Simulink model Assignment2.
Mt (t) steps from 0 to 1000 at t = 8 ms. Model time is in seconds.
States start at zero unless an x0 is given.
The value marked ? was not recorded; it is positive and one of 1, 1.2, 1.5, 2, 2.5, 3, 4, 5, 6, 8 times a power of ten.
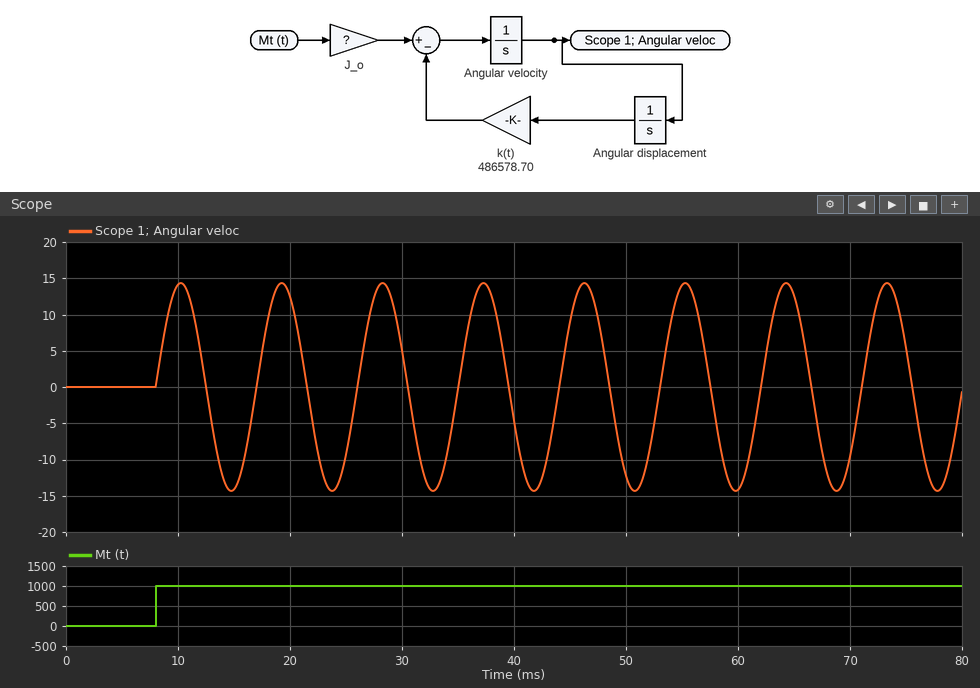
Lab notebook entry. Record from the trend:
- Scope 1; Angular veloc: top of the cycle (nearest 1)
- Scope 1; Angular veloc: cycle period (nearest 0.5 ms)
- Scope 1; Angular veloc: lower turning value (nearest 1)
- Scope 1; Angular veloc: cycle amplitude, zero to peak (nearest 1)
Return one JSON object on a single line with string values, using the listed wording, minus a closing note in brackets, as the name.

{"Scope 1; Angular veloc: top of the cycle": "14", "Scope 1; Angular veloc: cycle period": "9.0 ms", "Scope 1; Angular veloc: lower turning value": "-14", "Scope 1; Angular veloc: cycle amplitude, zero to peak": "14"}
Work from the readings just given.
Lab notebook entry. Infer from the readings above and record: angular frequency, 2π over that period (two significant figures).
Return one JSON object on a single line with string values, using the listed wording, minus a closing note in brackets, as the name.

{"angular frequency, 2π over that period": "0.70 rad/ms"}
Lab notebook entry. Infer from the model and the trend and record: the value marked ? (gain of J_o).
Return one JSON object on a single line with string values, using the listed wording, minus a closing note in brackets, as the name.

{"the value marked ?": "10"}
